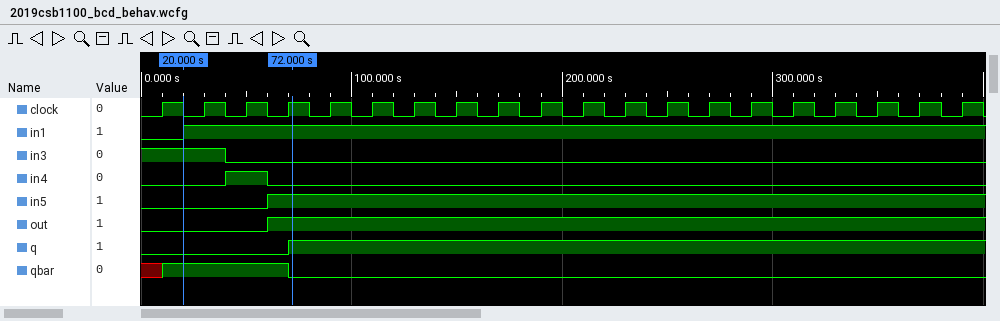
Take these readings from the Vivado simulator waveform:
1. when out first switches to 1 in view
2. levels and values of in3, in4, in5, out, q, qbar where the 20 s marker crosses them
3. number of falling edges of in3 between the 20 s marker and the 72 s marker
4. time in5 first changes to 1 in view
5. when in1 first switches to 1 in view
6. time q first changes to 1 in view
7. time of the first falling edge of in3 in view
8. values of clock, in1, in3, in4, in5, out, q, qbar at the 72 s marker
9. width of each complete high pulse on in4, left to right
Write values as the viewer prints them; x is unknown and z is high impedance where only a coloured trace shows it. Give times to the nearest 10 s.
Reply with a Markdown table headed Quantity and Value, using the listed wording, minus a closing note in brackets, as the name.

| Quantity | Value |
|---|---|
| when out first switches to 1 in view | 60 s |
| levels and values of in3, in4, in5, out, q, qbar where the 20 s marker crosses them | in3=1, in4=0, in5=0, out=0, q=0, qbar=1 |
| number of falling edges of in3 between the 20 s marker and the 72 s marker | 1 |
| time in5 first changes to 1 in view | 60 s |
| when in1 first switches to 1 in view | 20 s |
| time q first changes to 1 in view | 70 s |
| time of the first falling edge of in3 in view | 40 s |
| values of clock, in1, in3, in4, in5, out, q, qbar at the 72 s marker | clock=1, in1=1, in3=0, in4=0, in5=1, out=1, q=1, qbar=0 |
| width of each complete high pulse on in4, left to right | 20 s |
